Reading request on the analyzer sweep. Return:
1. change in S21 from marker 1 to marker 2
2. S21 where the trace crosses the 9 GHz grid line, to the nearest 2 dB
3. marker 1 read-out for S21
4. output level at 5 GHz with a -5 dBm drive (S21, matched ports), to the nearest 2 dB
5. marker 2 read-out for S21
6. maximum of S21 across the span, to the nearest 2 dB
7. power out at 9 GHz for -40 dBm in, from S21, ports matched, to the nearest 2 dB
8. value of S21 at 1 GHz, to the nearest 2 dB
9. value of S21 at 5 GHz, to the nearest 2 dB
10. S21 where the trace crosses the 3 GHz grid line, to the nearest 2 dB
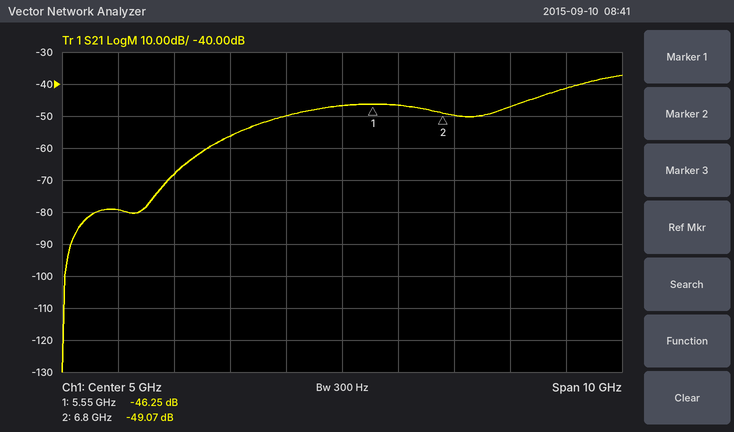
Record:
-2.82 dB
-42 dB
-46.25 dB
-52 dBm
-49.07 dB
-38 dB
-82 dBm
-80 dB
-46 dB
-56 dB
